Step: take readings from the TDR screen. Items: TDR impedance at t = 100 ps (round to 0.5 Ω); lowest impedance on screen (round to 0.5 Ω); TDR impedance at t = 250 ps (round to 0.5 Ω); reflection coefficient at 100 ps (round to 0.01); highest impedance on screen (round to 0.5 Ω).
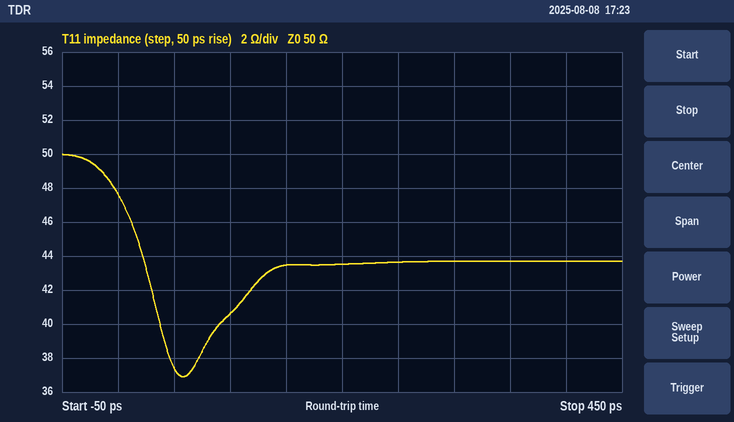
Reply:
40.5 Ω
37.0 Ω
43.5 Ω
-0.10
50.0 Ω
